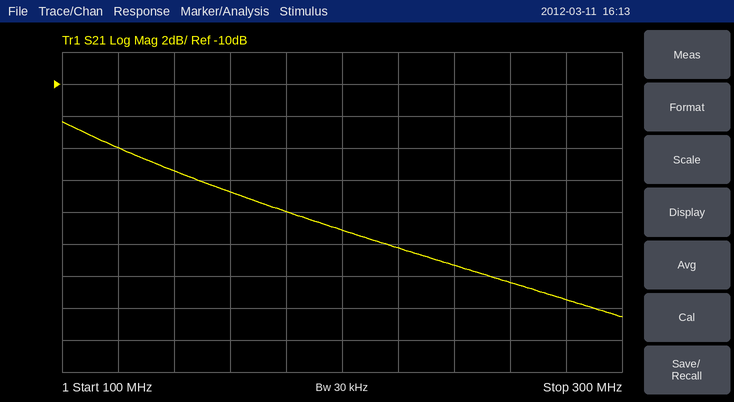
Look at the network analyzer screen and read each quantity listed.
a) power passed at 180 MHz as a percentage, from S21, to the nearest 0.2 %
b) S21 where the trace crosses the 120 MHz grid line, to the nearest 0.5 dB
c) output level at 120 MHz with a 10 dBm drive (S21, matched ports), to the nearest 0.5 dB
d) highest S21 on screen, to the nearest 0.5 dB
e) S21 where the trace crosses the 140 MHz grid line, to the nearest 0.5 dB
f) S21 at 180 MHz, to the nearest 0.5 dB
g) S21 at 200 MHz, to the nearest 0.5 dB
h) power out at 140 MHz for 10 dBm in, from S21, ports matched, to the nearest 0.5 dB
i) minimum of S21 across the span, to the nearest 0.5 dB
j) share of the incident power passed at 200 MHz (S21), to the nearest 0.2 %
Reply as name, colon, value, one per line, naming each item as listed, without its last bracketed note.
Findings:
power passed at 180 MHz as a percentage, from S21, to the nearest 0.2 %: 1.6 %
S21 where the trace crosses the 120 MHz grid line, to the nearest 0.5 dB: -14.0 dB
output level at 120 MHz with a 10 dBm drive (S21, matched ports), to the nearest 0.5 dB: -4.0 dBm
highest S21 on screen, to the nearest 0.5 dB: -12.5 dB
S21 where the trace crosses the 140 MHz grid line, to the nearest 0.5 dB: -15.5 dB
S21 at 180 MHz, to the nearest 0.5 dB: -18.0 dB
S21 at 200 MHz, to the nearest 0.5 dB: -19.0 dB
power out at 140 MHz for 10 dBm in, from S21, ports matched, to the nearest 0.5 dB: -5.5 dBm
minimum of S21 across the span, to the nearest 0.5 dB: -24.5 dB
share of the incident power passed at 200 MHz (S21), to the nearest 0.2 %: 1.2 %
